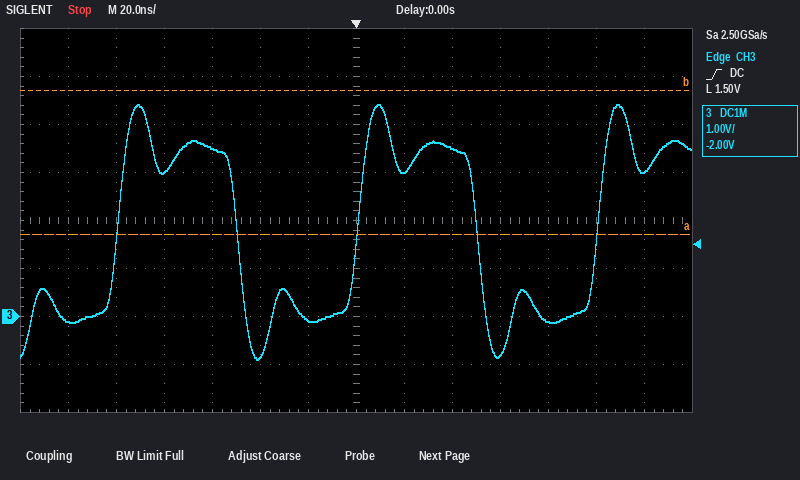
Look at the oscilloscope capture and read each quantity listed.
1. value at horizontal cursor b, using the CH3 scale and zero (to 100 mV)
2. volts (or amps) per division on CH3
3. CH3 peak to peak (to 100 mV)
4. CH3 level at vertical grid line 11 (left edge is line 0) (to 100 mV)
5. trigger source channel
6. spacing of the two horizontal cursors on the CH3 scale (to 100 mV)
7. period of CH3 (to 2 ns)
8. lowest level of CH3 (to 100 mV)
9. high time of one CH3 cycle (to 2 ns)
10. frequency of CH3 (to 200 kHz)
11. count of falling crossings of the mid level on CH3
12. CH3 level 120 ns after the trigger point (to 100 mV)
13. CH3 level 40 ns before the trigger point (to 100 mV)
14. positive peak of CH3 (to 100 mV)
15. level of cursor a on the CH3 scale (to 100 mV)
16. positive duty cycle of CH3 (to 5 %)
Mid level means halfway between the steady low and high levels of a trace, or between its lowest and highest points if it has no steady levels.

4.7 V
1 V
5.3 V
-100 mV
CH3
3.0 V
100 ns
-900 mV
50 ns
10.0 MHz
2
3.0 V
-800 mV
4.4 V
1.7 V
50 %
